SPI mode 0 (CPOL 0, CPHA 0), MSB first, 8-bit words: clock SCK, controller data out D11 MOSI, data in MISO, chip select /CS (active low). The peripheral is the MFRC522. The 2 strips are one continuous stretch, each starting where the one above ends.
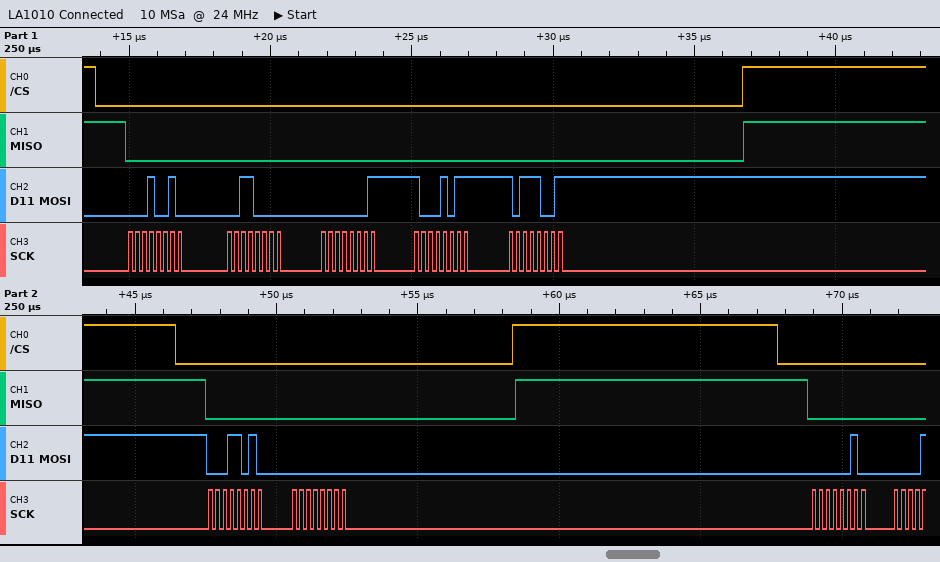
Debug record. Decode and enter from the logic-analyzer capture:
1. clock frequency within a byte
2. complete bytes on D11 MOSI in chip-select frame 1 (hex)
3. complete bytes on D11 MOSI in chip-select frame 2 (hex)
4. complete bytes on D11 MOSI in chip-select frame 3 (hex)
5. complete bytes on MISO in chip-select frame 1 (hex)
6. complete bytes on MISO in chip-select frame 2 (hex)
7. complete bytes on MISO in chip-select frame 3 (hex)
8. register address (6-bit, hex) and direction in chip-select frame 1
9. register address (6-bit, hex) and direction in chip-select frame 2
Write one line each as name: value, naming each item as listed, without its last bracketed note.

clock frequency within a byte: 4 MHz
complete bytes on D11 MOSI in chip-select frame 1: 12 30 01 8B B9
complete bytes on D11 MOSI in chip-select frame 2: 1A 00
complete bytes on D11 MOSI in chip-select frame 3: 02
complete bytes on MISO in chip-select frame 1: 00 00 00 00 00
complete bytes on MISO in chip-select frame 2: 00 00
complete bytes on MISO in chip-select frame 3: 00
register address (6-bit, hex) and direction in chip-select frame 1: 0x09 write
register address (6-bit, hex) and direction in chip-select frame 2: 0x0D write
